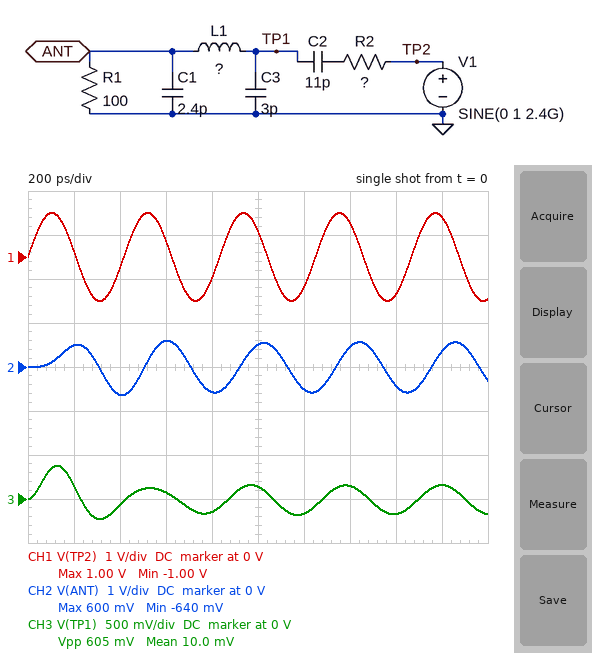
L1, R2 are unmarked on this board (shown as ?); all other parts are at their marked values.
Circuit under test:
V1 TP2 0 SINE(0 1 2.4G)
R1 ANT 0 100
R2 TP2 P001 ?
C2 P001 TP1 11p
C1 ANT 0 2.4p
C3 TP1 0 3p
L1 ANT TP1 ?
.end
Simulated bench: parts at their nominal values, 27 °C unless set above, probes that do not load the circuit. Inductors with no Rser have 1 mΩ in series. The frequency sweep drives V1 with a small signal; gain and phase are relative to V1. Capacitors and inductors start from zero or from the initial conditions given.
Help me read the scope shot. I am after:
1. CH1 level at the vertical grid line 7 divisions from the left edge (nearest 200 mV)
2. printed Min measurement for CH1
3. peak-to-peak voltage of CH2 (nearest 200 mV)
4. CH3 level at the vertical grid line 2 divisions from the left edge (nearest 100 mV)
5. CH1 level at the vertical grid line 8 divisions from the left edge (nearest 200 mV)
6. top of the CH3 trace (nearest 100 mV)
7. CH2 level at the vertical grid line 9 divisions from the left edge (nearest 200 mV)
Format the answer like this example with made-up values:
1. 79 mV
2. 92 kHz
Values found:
1. 800 mV
2. -1.00 V
3. 1.2 V
4. -100 mV
5. -800 mV
6. 400 mV
7. 400 mV
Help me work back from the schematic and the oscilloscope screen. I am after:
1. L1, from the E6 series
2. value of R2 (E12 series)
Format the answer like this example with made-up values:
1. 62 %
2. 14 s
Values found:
1. 1.5 nH
2. 33 Ω
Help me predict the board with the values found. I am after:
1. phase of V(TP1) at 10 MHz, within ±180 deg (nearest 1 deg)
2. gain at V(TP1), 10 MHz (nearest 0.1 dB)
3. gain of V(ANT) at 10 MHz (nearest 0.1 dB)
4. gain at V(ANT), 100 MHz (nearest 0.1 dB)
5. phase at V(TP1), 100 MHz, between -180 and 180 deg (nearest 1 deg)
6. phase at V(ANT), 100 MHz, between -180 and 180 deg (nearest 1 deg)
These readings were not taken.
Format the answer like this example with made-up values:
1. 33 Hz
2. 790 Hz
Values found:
1. 83 deg
2. -23.3 dB
3. -23.3 dB
4. -7.0 dB
5. 37 deg
6. 36 deg
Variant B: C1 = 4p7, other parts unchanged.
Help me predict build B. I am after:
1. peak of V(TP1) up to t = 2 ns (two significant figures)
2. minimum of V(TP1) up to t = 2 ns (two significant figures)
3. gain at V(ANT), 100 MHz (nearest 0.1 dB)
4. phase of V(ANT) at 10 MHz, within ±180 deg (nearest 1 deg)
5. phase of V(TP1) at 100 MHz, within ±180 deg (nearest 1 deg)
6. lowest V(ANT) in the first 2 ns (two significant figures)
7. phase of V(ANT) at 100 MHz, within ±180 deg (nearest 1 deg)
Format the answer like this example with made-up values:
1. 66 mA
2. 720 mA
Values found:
1. 410 mV
2. -440 mV
3. -7.6 dB
4. 82 deg
5. 33 deg
6. -610 mV
7. 32 deg
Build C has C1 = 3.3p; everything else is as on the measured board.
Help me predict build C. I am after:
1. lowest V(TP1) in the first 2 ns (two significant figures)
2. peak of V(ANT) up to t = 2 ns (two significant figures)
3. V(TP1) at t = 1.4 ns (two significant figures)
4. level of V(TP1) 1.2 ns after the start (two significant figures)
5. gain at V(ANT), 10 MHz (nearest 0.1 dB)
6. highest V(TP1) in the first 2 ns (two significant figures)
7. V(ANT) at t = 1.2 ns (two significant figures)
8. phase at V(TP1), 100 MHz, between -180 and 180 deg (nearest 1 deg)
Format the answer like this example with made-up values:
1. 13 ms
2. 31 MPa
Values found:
1. -280 mV
2. 620 mV
3. 38 mV
4. -37 mV
5. -23.3 dB
6. 370 mV
7. -480 mV
8. 35 deg
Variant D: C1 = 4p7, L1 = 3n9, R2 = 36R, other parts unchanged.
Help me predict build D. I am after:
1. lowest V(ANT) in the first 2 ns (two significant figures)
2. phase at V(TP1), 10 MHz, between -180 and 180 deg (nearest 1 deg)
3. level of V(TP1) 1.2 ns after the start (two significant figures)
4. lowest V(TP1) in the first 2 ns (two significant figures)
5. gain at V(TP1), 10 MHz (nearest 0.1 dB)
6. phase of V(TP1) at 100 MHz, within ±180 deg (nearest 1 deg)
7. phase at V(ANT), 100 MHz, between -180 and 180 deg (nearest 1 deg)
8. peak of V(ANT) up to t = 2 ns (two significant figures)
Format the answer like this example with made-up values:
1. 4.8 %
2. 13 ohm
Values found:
1. -330 mV
2. 82 deg
3. -690 mV
4. -780 mV
5. -23.3 dB
6. 33 deg
7. 31 deg
8. 300 mV
